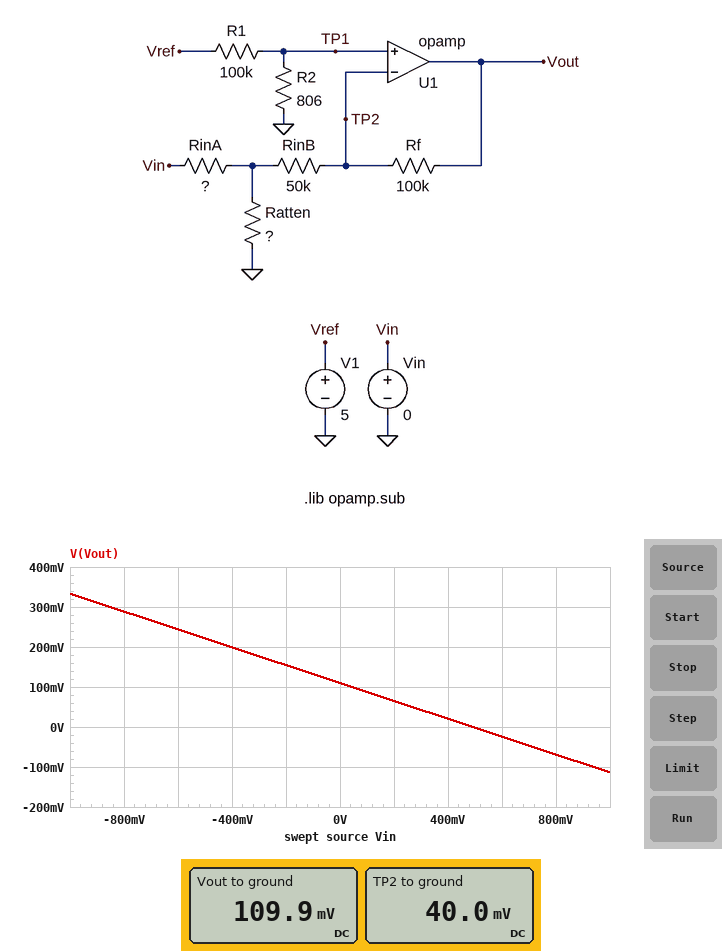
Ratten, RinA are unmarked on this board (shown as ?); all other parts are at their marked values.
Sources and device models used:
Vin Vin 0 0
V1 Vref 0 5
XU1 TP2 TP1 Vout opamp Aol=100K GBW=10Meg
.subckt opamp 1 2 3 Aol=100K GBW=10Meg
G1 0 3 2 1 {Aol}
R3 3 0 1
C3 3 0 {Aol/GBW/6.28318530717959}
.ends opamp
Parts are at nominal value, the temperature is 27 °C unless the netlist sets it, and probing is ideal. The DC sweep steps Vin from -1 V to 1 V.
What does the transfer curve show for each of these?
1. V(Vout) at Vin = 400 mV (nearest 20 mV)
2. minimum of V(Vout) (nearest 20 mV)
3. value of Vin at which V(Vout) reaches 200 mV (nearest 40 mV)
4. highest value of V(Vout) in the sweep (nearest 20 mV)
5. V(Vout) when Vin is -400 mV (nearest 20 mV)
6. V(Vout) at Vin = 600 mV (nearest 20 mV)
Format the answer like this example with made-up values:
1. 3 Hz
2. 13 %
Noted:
1. 20 mV
2. -120 mV
3. -400 mV
4. 340 mV
5. 200 mV
6. -20 mV
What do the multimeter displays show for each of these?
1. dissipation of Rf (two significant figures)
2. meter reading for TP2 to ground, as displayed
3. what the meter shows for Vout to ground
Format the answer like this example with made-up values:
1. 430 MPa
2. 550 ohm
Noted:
1. 49 nW
2. 40.0 mV
3. 109.9 mV
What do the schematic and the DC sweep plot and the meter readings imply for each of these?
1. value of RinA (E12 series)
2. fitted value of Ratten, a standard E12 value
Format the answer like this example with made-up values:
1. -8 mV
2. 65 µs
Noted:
1. 56 kΩ
2. 8.2 kΩ
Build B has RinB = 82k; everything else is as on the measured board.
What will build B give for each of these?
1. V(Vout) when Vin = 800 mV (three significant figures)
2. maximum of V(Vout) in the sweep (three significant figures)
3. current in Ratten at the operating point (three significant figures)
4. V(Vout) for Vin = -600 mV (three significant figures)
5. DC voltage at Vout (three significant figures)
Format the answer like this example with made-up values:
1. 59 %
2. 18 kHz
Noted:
1. -29.8 mV
2. 228 mV
3. 391 nA
4. 171 mV
5. 84.8 mV
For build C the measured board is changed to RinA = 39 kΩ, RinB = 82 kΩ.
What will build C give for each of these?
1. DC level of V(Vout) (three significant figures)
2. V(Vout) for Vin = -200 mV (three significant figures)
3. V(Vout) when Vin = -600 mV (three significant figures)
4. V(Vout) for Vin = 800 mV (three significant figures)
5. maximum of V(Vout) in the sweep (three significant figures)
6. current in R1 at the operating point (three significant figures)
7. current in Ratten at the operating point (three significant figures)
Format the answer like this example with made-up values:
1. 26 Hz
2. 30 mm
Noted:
1. 85.0 mV
2. 124 mV
3. 202 mV
4. -71.5 mV
5. 281 mV
6. 49.6 µA
7. 372 nA
